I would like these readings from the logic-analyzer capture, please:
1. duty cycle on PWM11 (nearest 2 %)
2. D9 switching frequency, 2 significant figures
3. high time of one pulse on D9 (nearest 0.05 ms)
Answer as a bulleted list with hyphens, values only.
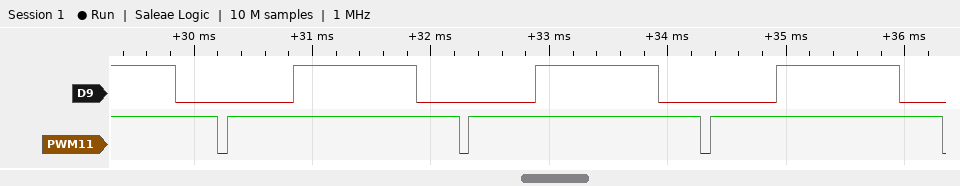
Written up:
- 96 %
- 490 Hz
- 1.05 ms
